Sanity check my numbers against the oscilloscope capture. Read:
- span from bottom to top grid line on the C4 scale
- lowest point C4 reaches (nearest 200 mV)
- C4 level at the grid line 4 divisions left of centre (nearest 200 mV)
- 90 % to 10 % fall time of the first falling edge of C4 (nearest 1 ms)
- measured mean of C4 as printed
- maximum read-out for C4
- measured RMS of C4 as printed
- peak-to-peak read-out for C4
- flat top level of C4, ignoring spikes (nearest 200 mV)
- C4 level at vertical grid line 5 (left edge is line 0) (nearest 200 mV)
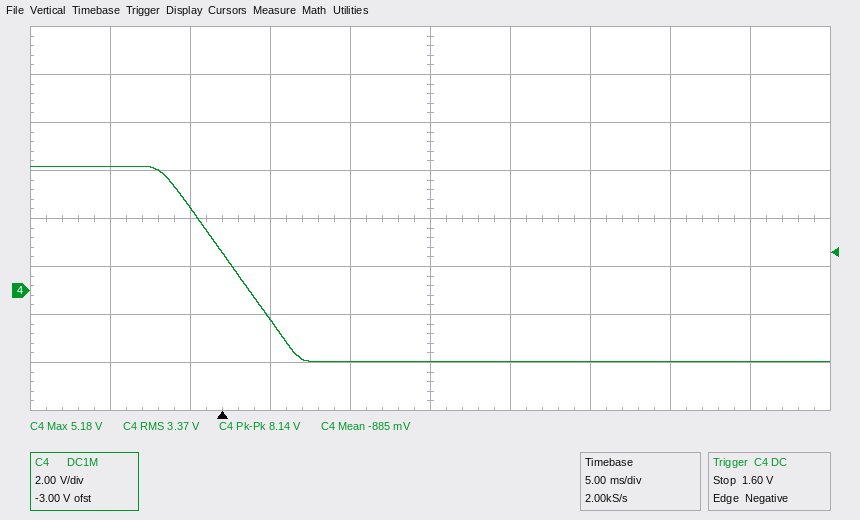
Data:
16 V
-3.0 V
5.2 V
7 ms
-885 mV
5.18 V
3.37 V
8.14 V
5.2 V
-3.0 V
